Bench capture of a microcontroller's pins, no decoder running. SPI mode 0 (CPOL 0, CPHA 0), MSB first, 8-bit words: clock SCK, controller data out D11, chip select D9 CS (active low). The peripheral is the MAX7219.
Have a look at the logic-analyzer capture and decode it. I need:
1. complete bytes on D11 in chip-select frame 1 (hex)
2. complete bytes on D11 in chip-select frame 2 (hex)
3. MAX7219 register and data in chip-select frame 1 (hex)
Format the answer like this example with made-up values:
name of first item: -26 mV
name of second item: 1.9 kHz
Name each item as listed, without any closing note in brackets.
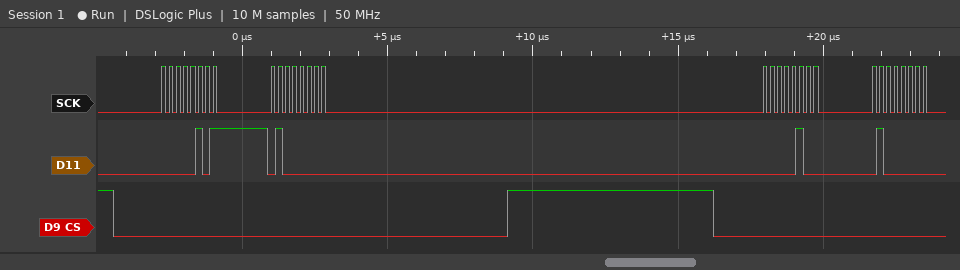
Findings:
complete bytes on D11 in chip-select frame 1: 05 40
complete bytes on D11 in chip-select frame 2: 04 40
MAX7219 register and data in chip-select frame 1: register 0x5, data 0x40
